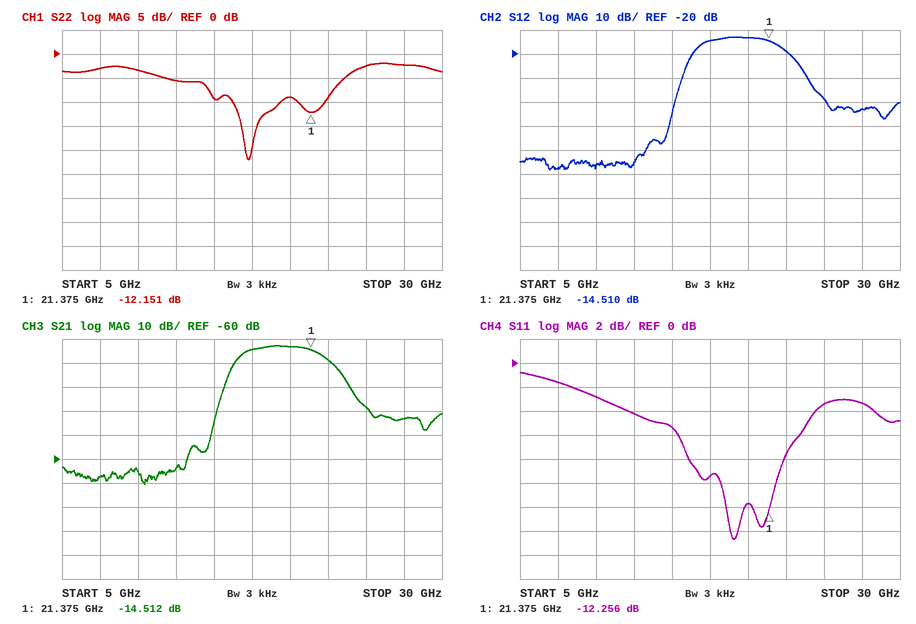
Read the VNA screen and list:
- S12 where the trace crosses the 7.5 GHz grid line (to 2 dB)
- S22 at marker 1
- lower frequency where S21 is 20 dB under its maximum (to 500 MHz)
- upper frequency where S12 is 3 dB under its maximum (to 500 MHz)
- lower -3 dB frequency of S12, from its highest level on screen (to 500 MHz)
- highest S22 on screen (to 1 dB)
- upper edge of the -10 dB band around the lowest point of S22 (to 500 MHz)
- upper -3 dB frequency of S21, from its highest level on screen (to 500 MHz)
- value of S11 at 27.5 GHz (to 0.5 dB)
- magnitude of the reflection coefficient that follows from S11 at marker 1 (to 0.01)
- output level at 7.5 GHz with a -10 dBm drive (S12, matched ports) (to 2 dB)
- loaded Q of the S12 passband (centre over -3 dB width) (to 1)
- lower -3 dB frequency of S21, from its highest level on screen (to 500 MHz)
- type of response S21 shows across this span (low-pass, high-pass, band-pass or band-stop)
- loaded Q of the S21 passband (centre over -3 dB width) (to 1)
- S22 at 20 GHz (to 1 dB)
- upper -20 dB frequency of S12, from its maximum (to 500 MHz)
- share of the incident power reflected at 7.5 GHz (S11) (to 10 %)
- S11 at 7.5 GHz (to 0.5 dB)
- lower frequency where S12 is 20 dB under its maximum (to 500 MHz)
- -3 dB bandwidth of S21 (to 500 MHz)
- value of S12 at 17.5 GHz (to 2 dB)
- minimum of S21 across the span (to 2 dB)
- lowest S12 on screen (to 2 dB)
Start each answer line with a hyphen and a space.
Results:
- -68 dB
- -12.151 dB
- 15.5 GHz
- 22.0 GHz
- 17.0 GHz
- -2 dB
- 19.5 GHz
- 22.0 GHz
- -3.5 dB
- 0.24
- -78 dBm
- 4
- 17.0 GHz
- band-pass
- 4
- -9 dB
- 24.0 GHz
- 70 %
- -1.5 dB
- 15.5 GHz
- 5.0 GHz
- -14 dB
- -70 dB
- -68 dB
